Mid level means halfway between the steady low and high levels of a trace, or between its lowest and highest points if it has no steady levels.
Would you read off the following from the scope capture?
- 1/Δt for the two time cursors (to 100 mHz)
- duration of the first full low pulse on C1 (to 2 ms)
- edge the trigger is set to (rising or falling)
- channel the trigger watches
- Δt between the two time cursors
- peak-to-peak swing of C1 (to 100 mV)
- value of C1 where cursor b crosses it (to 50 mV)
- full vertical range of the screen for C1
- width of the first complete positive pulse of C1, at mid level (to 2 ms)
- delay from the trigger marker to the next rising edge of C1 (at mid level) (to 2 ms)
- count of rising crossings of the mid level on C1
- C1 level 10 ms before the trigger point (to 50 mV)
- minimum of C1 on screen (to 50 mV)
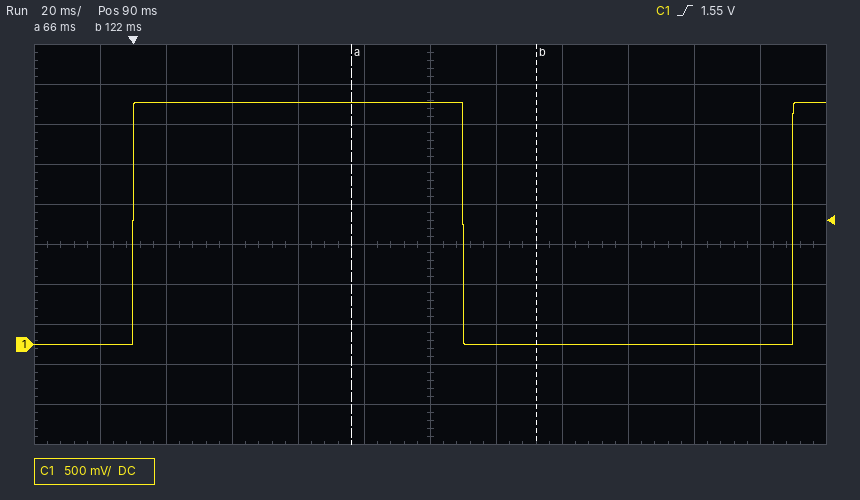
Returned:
17.9 Hz
100 ms
rising
C1
56 ms
3.00 V
0 mV
5 V
100 ms
200 ms
2
0 mV
0 mV
